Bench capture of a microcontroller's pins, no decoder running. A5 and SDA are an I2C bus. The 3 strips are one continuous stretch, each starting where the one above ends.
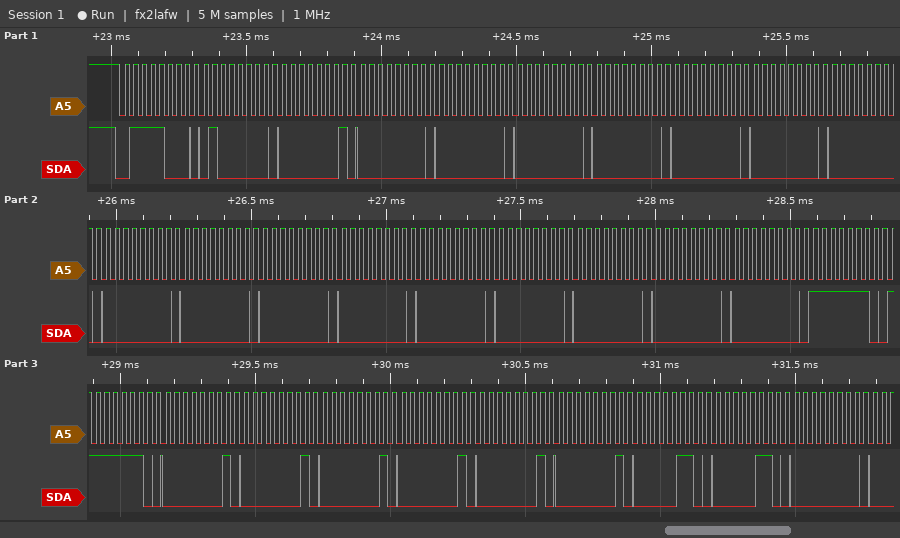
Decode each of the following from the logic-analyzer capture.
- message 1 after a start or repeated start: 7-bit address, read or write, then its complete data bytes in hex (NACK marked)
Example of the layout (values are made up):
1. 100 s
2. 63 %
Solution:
1. 0x3C write: 40 01 00 00 00 00 00 00 00 00 00 00 00 00 00 00 00 00 FE FE 01 01 01 01 01 01 06 06 00
